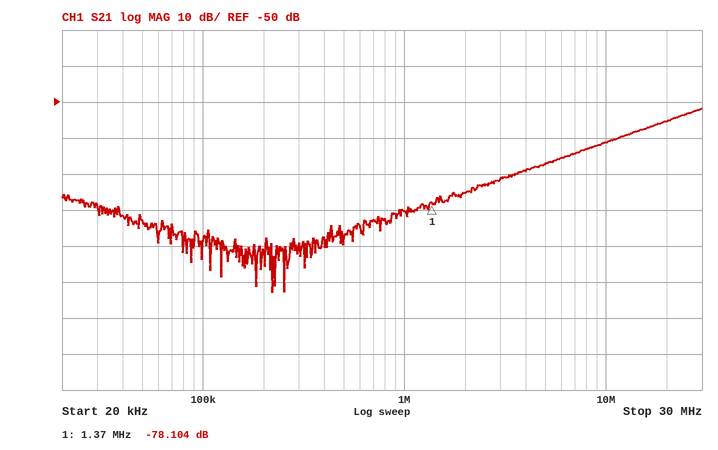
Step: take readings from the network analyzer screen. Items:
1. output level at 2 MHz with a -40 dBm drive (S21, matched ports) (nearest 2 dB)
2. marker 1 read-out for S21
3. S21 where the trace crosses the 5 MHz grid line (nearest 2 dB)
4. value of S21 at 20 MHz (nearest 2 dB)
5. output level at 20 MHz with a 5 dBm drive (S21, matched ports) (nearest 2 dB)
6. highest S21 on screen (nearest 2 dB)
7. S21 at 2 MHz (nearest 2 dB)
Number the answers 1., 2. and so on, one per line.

1. -116 dBm
2. -78.104 dB
3. -68 dB
4. -56 dB
5. -50 dBm
6. -52 dB
7. -76 dB
